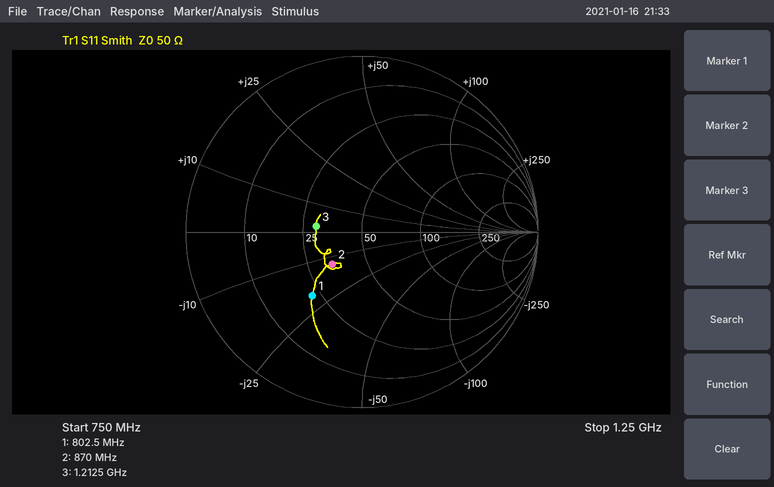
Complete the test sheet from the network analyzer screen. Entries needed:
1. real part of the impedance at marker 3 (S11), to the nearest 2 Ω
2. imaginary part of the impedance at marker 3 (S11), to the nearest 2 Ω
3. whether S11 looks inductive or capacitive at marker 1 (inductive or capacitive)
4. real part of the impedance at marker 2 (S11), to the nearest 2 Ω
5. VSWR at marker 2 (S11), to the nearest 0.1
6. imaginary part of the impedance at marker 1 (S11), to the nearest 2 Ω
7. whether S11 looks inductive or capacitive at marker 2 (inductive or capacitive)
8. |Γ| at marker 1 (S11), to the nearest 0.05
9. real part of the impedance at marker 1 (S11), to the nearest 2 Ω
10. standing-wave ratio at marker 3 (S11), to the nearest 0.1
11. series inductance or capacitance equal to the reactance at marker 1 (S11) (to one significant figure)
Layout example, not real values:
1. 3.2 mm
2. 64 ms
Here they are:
1. 30 Ω
2. +2 Ω
3. capacitive
4. 34 Ω
5. 1.7
6. -20 Ω
7. capacitive
8. 0.45
9. 22 Ω
10. 1.7
11. 10 pF
